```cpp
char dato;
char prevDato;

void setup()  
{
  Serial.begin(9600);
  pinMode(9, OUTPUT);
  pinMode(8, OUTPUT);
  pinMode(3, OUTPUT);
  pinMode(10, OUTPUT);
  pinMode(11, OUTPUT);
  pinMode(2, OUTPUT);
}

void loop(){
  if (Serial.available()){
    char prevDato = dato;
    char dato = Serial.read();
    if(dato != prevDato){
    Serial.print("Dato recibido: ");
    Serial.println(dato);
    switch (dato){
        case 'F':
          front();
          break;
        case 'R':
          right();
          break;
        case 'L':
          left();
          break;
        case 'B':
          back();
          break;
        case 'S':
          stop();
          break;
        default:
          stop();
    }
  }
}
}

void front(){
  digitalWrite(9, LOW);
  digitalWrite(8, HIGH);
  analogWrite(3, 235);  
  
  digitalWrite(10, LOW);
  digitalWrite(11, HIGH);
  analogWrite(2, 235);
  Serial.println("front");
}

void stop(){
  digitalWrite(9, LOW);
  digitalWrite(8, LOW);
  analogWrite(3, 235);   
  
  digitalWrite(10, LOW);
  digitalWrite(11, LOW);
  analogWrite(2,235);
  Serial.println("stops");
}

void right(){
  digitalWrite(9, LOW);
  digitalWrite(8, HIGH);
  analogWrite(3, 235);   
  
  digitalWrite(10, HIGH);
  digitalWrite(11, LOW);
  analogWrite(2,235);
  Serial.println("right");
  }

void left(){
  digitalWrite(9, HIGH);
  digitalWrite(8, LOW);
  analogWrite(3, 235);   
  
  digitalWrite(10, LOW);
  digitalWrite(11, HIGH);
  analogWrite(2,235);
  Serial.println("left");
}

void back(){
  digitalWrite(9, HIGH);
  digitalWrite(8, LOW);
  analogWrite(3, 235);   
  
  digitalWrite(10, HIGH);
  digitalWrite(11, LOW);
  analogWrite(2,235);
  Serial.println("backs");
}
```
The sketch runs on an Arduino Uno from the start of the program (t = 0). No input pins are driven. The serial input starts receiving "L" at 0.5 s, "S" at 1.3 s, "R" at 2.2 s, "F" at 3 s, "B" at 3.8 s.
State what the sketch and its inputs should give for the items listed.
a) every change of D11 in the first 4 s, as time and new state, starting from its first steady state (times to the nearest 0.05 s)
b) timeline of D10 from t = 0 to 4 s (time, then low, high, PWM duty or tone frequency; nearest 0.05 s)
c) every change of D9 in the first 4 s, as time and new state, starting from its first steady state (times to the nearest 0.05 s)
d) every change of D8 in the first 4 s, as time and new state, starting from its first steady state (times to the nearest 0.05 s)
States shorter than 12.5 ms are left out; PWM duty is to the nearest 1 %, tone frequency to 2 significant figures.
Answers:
0 s low; 0.5 s high; 1.3 s low; 3 s high; 3.8 s low
0 s low; 2.2 s high; 3 s low; 3.8 s high
0 s low; 0.5 s high; 1.3 s low; 3.8 s high
0 s low; 2.2 s high; 3.8 s low
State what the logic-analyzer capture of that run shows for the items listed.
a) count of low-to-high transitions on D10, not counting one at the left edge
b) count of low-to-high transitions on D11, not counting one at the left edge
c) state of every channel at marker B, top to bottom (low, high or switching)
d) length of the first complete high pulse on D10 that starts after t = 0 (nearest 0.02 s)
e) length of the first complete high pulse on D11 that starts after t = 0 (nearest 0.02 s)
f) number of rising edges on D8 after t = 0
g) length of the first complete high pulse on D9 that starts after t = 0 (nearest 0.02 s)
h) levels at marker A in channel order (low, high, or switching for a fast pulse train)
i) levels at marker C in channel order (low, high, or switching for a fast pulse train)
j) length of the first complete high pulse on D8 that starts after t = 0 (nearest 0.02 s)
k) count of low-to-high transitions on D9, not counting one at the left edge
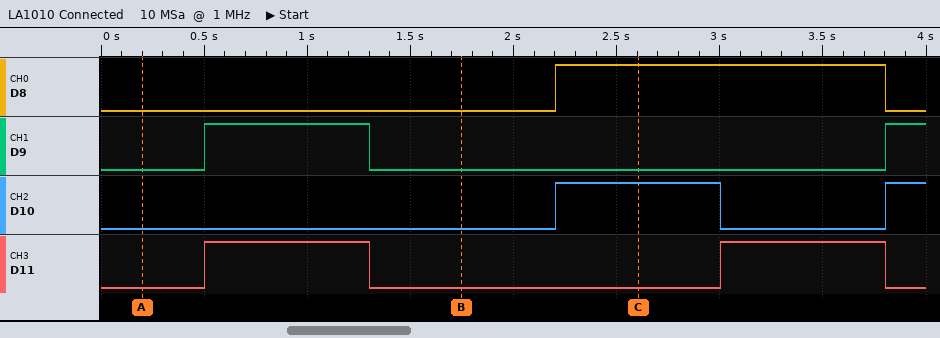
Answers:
2
2
D8 low, D9 low, D10 low, D11 low
0.80 s
0.80 s
1
0.80 s
D8 low, D9 low, D10 low, D11 low
D8 high, D9 low, D10 high, D11 low
1.60 s
2
